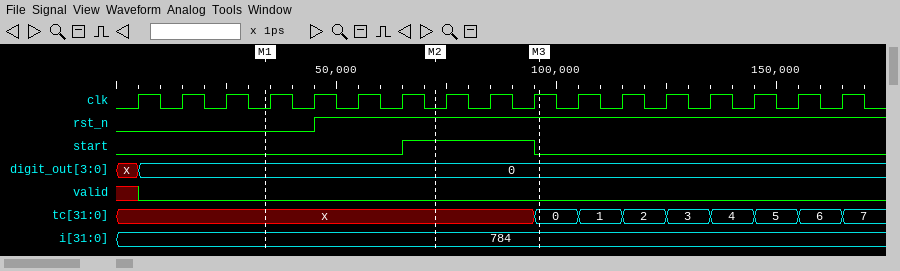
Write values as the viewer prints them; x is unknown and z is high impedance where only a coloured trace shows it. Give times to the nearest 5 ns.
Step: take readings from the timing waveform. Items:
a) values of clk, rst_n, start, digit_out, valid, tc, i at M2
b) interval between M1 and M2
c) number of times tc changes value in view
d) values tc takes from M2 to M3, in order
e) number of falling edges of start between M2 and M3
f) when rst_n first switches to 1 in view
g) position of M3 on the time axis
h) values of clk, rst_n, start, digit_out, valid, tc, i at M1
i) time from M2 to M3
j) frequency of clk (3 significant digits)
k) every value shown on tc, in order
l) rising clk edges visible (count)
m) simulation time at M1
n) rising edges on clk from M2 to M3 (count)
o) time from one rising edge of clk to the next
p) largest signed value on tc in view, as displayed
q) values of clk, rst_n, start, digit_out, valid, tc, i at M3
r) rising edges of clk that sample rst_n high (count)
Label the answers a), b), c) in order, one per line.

a) clk=0, rst_n=1, start=1, digit_out=0, valid=0, tc=x, i=784
b) 40 ns
c) 8
d) x, 0
e) 1
f) 45 ns
g) 95 ns
h) clk=0, rst_n=0, start=0, digit_out=0, valid=0, tc=x, i=784
i) 25 ns
j) 100 MHz
k) x, 0, 1, 2, 3, 4, 5, 6, 7
l) 17
m) 35 ns
n) 3
o) 10 ns
p) 7
q) clk=1, rst_n=1, start=0, digit_out=0, valid=0, tc=0, i=784
r) 12
